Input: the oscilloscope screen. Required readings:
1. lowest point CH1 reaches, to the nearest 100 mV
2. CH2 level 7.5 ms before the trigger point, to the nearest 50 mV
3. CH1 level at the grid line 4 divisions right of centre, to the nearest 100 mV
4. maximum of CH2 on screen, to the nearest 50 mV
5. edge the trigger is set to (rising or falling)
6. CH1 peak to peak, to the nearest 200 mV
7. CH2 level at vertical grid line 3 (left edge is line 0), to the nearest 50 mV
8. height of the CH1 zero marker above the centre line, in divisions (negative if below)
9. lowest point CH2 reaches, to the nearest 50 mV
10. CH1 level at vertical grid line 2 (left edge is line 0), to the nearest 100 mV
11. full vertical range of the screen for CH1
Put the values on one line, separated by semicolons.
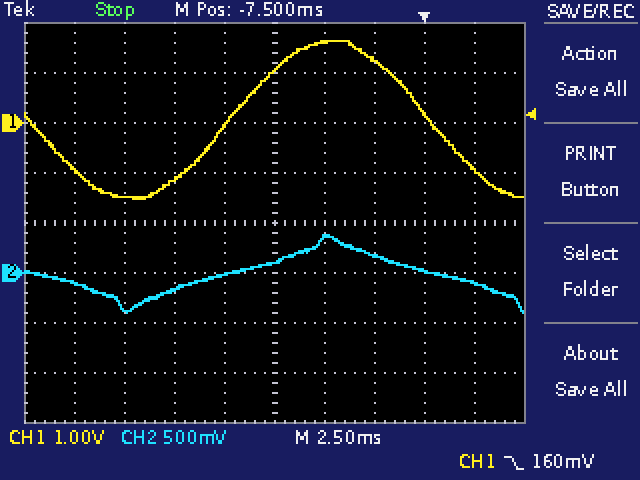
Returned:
-1.5 V; 100 mV; -900 mV; 400 mV; falling; 3.2 V; -150 mV; +2.0 div; -400 mV; -1.5 V; 8 V
